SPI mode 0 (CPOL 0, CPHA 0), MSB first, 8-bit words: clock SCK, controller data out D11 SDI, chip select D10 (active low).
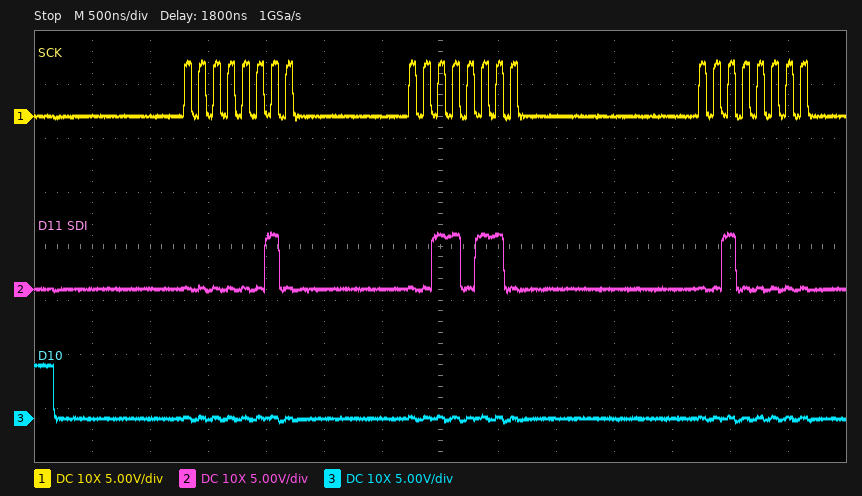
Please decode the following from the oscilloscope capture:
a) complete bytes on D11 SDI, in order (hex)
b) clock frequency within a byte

0x02 0x36 0x20
8 MHz
